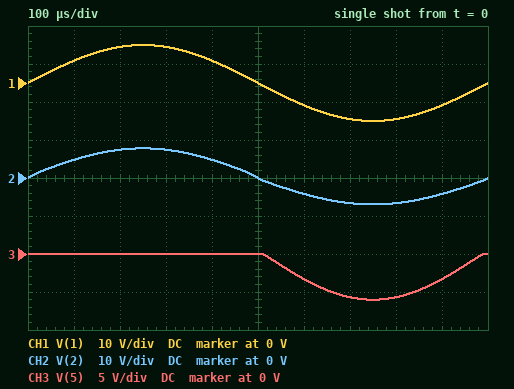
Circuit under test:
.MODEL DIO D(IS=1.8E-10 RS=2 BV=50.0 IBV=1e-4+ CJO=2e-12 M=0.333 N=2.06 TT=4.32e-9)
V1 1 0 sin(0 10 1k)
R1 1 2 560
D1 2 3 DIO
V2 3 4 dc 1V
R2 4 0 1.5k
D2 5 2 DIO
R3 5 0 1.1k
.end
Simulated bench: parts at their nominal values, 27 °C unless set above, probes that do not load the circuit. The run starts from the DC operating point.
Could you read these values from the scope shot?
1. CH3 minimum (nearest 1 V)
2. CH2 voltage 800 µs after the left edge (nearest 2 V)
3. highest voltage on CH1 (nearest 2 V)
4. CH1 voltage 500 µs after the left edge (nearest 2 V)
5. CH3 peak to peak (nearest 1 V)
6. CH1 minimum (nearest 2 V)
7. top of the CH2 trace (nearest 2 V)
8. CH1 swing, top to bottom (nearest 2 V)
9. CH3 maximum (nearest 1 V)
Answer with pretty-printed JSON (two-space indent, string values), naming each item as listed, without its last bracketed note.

{
  "CH3 minimum": "-6 V",
  "CH2 voltage 800 µs after the left edge": "-6 V",
  "highest voltage on CH1": "10 V",
  "CH1 voltage 500 µs after the left edge": "0 V",
  "CH3 peak to peak": "6 V",
  "CH1 minimum": "-10 V",
  "top of the CH2 trace": "8 V",
  "CH1 swing, top to bottom": "20 V",
  "CH3 maximum": "0 V"
}
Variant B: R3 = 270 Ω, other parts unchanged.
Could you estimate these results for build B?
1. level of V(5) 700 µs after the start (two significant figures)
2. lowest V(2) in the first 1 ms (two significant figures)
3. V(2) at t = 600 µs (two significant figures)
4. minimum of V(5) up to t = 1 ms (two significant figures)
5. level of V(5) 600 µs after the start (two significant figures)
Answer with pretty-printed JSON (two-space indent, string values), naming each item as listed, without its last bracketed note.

{
  "level of V(5) 700 µs after the start": "-2.8 V",
  "lowest V(2) in the first 1 ms": "-3.9 V",
  "V(2) at t = 600 µs": "-2.5 V",
  "minimum of V(5) up to t = 1 ms": "-2.9 V",
  "level of V(5) 600 µs after the start": "-1.6 V"
}
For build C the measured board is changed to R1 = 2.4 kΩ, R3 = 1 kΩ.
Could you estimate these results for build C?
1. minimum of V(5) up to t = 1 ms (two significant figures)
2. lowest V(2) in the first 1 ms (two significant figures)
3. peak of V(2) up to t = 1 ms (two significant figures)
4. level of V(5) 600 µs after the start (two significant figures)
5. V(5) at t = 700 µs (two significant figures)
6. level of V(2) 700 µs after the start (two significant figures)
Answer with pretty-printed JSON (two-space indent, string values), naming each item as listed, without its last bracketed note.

{
  "minimum of V(5) up to t = 1 ms": "-2.7 V",
  "lowest V(2) in the first 1 ms": "-3.6 V",
  "peak of V(2) up to t = 1 ms": "5.0 V",
  "level of V(5) 600 µs after the start": "-1.5 V",
  "V(5) at t = 700 µs": "-2.5 V",
  "level of V(2) 700 µs after the start": "-3.4 V"
}
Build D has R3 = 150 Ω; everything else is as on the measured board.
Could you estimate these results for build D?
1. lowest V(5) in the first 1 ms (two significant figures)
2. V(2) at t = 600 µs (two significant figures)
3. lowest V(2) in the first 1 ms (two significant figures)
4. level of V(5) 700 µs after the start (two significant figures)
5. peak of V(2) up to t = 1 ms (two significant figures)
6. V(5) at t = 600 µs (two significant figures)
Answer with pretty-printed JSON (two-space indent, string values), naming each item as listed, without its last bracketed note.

{
  "lowest V(5) in the first 1 ms": "-1.9 V",
  "V(2) at t = 600 µs": "-2.0 V",
  "lowest V(2) in the first 1 ms": "-2.9 V",
  "level of V(5) 700 µs after the start": "-1.8 V",
  "peak of V(2) up to t = 1 ms": "7.8 V",
  "V(5) at t = 600 µs": "-1.0 V"
}
